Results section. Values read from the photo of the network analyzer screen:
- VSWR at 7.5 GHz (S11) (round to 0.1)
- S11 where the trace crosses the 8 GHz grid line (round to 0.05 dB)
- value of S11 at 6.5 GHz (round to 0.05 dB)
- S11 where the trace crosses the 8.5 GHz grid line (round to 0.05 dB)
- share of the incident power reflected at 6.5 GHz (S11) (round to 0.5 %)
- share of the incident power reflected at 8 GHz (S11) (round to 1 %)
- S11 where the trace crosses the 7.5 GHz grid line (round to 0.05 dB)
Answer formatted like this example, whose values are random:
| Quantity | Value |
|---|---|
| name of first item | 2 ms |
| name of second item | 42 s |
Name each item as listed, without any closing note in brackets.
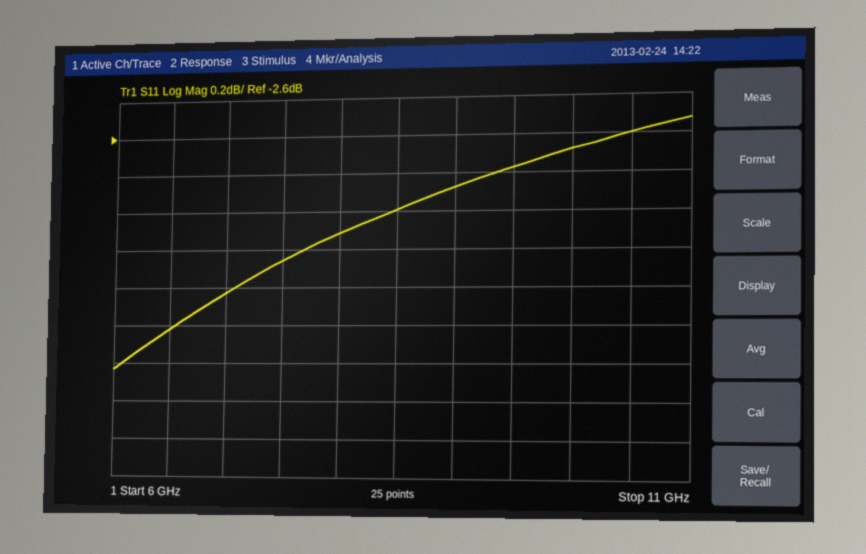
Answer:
| Quantity | Value |
|---|---|
| VSWR at 7.5 GHz (S11) | 5.4 |
| S11 where the trace crosses the 8 GHz grid line | -3.10 dB |
| value of S11 at 6.5 GHz | -3.60 dB |
| S11 where the trace crosses the 8.5 GHz grid line | -3.00 dB |
| share of the incident power reflected at 6.5 GHz (S11) | 43.5 % |
| share of the incident power reflected at 8 GHz (S11) | 49 % |
| S11 where the trace crosses the 7.5 GHz grid line | -3.25 dB |
